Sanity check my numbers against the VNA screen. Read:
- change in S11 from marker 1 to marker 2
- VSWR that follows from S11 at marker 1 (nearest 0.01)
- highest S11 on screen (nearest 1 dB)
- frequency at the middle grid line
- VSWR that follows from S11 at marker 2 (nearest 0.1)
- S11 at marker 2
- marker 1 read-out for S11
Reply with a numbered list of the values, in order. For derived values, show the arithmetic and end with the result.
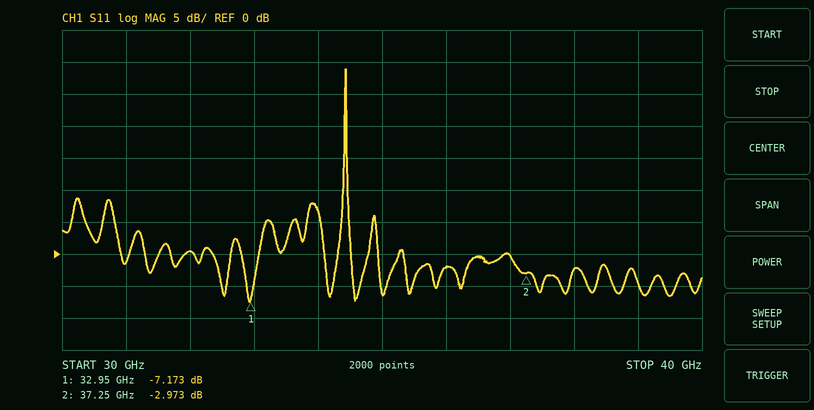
1. -2.973 − (-7.173) = 4.200 dB
2. (1 + 0.4379)/(1 − 0.4379) ≈ 2.56
3. 29 dB
4. 35 GHz
5. (1 + 0.7101)/(1 − 0.7101) ≈ 5.9
6. -2.973 dB
7. -7.173 dB
